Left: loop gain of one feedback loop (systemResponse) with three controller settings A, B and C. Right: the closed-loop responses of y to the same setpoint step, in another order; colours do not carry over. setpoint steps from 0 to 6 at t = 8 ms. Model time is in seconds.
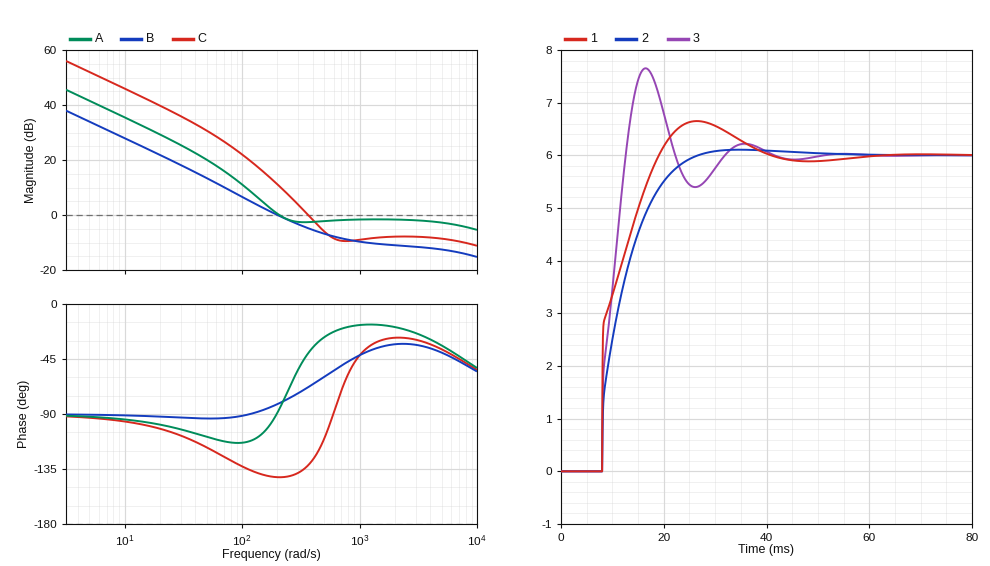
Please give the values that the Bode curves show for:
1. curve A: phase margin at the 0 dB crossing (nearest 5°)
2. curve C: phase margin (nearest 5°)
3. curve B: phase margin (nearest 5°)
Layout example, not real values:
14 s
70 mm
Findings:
95°
50°
100°
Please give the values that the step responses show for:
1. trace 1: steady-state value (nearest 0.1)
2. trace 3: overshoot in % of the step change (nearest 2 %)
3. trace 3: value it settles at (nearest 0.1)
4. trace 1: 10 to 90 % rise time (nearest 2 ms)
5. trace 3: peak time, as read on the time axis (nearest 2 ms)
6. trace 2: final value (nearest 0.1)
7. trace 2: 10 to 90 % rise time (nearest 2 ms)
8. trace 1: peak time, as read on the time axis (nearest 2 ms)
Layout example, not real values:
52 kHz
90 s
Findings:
6.0
28 %
6.0
8 ms
16 ms
6.0
12 ms
26 ms
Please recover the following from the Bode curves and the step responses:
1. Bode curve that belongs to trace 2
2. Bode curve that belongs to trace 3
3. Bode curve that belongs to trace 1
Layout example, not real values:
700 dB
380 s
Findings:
B
C
A
